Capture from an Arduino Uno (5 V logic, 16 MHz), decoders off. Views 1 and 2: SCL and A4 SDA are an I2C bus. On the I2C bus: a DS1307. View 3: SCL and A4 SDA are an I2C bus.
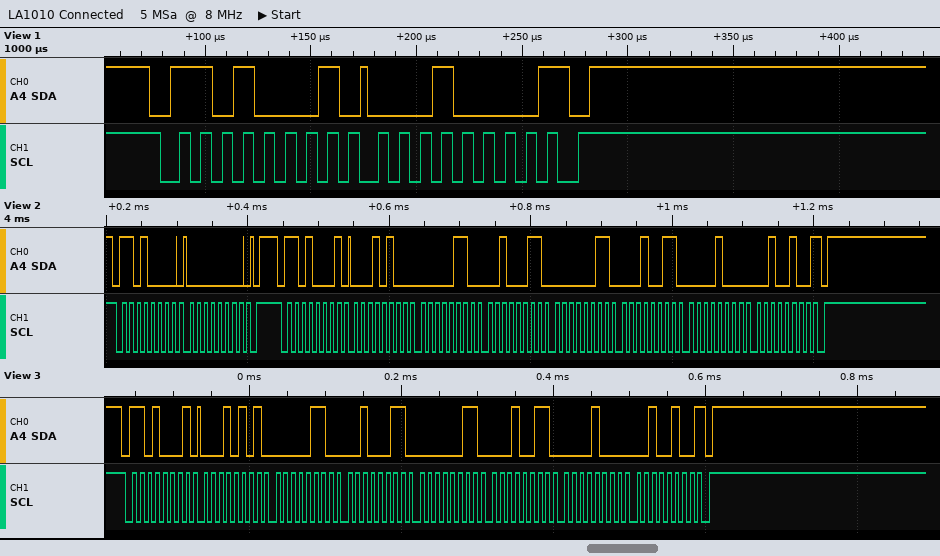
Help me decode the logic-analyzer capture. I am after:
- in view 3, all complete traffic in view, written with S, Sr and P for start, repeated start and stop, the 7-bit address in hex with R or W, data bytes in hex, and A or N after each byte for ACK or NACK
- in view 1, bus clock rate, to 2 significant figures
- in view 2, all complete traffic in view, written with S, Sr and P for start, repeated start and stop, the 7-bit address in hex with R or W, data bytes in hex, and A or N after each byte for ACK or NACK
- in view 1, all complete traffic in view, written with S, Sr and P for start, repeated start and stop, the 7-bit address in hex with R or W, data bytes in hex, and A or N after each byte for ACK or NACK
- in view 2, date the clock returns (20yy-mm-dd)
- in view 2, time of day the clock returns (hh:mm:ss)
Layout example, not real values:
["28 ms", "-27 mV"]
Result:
["S 68R A 15 A 06 A 23 A 03 A 13 A 08 A 24 N P", "100 kHz", "S 68W A 00 A P S 68R A 14 A 06 A 23 A 03 A 13 A 08 A 24 N P", "S 68R A 10 N P", "2024-08-13", "23:06:14"]
